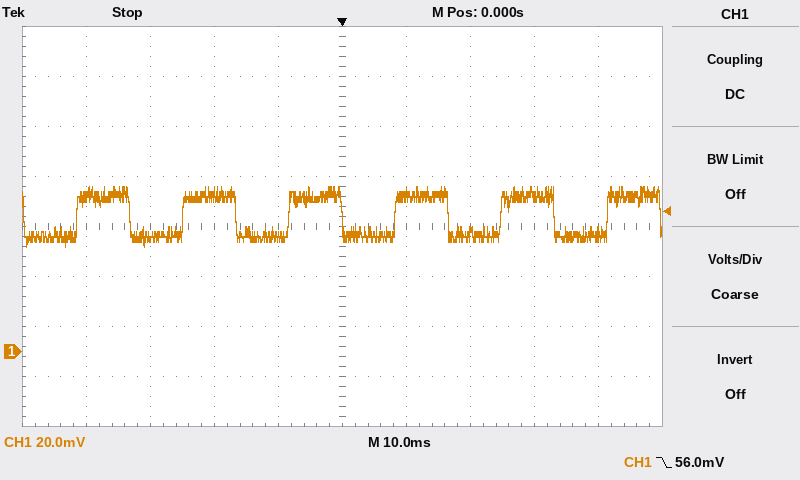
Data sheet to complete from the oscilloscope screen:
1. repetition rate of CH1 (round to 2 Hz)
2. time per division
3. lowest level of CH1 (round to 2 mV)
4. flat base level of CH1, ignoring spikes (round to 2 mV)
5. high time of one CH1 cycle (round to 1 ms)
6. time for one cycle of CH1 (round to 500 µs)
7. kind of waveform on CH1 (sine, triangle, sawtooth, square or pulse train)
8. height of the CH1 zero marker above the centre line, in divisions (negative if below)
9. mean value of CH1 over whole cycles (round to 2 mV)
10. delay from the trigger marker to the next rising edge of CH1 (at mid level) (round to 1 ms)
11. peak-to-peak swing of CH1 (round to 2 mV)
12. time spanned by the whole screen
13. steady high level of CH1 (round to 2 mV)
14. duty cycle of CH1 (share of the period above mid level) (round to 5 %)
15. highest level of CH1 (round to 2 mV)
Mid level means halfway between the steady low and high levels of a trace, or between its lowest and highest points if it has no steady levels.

60 Hz
10 ms
42 mV
46 mV
8 ms
16.5 ms
square
-2.5 div
54 mV
8 ms
24 mV
100 ms
62 mV
50 %
66 mV
